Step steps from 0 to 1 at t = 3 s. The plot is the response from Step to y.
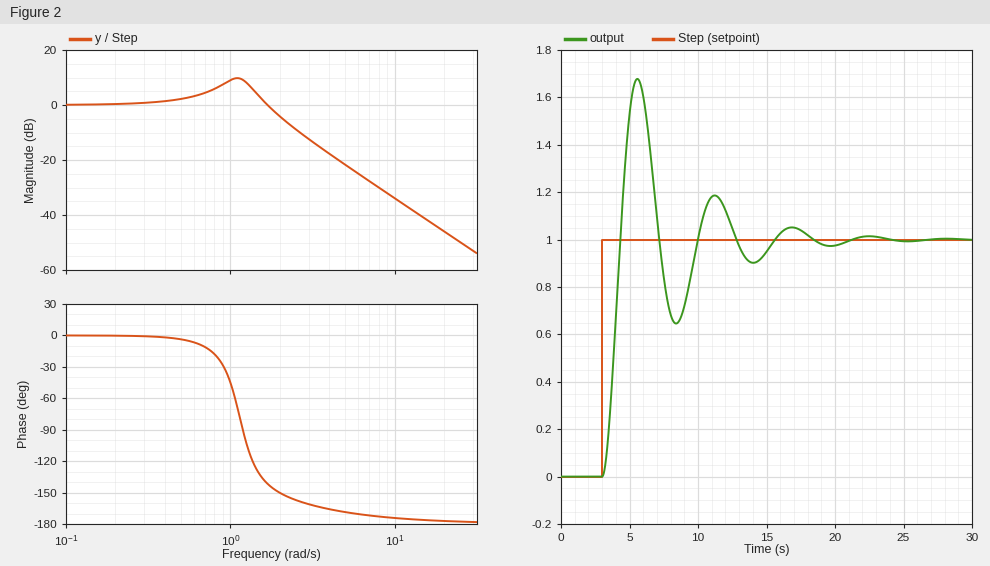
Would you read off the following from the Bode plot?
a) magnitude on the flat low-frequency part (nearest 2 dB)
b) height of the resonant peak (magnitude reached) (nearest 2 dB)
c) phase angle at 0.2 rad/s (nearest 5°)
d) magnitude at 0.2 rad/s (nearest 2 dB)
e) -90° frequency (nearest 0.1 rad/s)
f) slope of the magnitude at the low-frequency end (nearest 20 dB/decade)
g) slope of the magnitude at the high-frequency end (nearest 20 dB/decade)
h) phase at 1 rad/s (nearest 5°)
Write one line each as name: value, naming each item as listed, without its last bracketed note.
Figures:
magnitude on the flat low-frequency part: 0 dB
height of the resonant peak (magnitude reached): 10 dB
phase angle at 0.2 rad/s: 0°
magnitude at 0.2 rad/s: 0 dB
-90° frequency: 1.2 rad/s
slope of the magnitude at the low-frequency end: 0 dB/decade
slope of the magnitude at the high-frequency end: -40 dB/decade
phase at 1 rad/s: -45°
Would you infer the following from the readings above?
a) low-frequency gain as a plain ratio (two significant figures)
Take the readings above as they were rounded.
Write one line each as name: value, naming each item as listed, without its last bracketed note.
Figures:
low-frequency gain as a plain ratio: 1.0
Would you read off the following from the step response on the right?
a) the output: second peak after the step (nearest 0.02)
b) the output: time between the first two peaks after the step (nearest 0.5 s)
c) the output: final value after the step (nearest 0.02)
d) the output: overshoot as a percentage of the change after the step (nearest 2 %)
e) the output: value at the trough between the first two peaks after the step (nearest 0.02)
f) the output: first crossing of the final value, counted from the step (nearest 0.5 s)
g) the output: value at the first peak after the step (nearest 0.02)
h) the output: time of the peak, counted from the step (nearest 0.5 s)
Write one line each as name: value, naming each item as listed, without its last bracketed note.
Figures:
the output: second peak after the step: 1.18
the output: time between the first two peaks after the step: 5.5 s
the output: final value after the step: 1.00
the output: overshoot as a percentage of the change after the step: 68 %
the output: value at the trough between the first two peaks after the step: 0.64
the output: first crossing of the final value, counted from the step: 1.5 s
the output: value at the first peak after the step: 1.68
the output: time of the peak, counted from the step: 2.5 s
